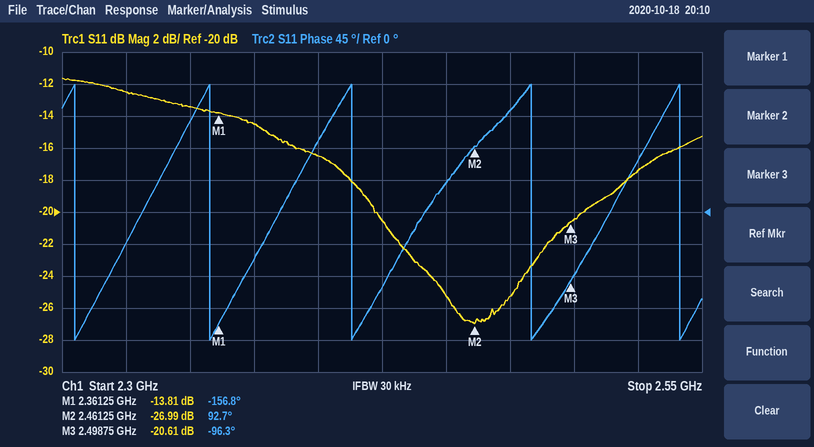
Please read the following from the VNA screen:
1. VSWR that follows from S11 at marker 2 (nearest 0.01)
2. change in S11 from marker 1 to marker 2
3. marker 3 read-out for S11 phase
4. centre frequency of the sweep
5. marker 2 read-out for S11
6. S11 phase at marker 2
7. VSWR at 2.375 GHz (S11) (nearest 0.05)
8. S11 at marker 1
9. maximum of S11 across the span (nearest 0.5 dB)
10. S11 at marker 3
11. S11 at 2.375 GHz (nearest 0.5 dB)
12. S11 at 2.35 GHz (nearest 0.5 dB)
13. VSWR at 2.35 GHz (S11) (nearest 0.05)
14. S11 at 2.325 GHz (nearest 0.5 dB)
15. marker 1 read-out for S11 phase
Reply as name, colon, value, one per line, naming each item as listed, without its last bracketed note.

VSWR that follows from S11 at marker 2: 1.09
change in S11 from marker 1 to marker 2: -13.18 dB
marker 3 read-out for S11 phase: -96.3°
centre frequency of the sweep: 2.425 GHz
marker 2 read-out for S11: -26.99 dB
S11 phase at marker 2: 92.7°
VSWR at 2.375 GHz (S11): 1.45
S11 at marker 1: -13.81 dB
maximum of S11 across the span: -11.5 dB
S11 at marker 3: -20.61 dB
S11 at 2.375 GHz: -14.5 dB
S11 at 2.35 GHz: -13.5 dB
VSWR at 2.35 GHz (S11): 1.55
S11 at 2.325 GHz: -12.5 dB
marker 1 read-out for S11 phase: -156.8°
